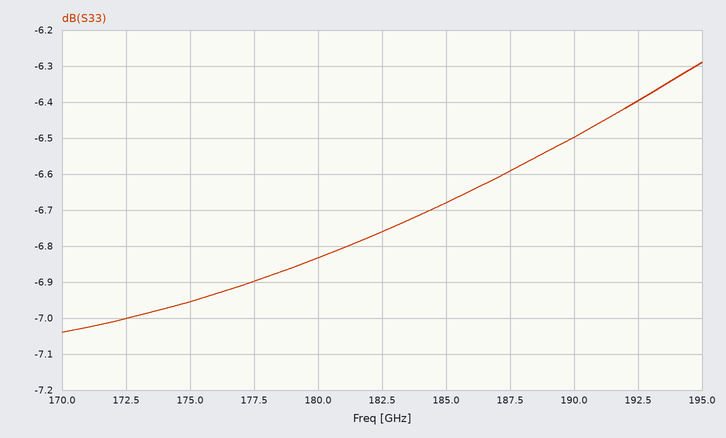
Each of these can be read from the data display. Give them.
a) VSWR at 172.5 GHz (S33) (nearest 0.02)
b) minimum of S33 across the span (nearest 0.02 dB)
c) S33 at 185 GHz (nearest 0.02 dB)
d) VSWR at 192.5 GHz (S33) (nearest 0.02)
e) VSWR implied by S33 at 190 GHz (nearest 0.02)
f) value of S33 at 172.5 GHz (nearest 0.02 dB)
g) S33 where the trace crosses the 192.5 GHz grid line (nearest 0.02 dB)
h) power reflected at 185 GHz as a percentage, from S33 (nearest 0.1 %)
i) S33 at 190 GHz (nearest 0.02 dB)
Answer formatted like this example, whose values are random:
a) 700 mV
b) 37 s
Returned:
a) 2.62
b) -7.04 dB
c) -6.68 dB
d) 2.84
e) 2.80
f) -7.00 dB
g) -6.40 dB
h) 21.5 %
i) -6.50 dB
